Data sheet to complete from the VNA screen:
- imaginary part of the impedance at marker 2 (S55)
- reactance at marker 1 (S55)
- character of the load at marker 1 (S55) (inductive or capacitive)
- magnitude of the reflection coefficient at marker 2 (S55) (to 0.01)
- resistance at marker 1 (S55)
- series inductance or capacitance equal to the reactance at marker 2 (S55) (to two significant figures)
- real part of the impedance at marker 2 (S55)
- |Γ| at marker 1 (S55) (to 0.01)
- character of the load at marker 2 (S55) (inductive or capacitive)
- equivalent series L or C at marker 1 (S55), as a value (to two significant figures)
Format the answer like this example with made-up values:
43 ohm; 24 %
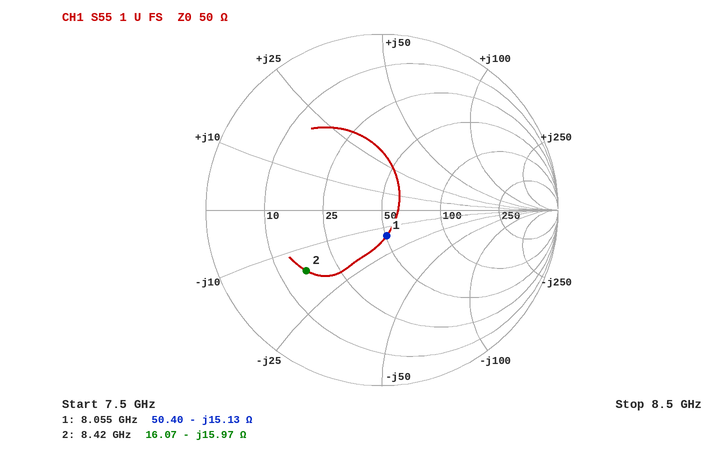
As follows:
-15.97 Ω; -15.13 Ω; capacitive; 0.55; 50.40 Ω; 1.2 pF; 16.07 Ω; 0.15; capacitive; 1.3 pF
